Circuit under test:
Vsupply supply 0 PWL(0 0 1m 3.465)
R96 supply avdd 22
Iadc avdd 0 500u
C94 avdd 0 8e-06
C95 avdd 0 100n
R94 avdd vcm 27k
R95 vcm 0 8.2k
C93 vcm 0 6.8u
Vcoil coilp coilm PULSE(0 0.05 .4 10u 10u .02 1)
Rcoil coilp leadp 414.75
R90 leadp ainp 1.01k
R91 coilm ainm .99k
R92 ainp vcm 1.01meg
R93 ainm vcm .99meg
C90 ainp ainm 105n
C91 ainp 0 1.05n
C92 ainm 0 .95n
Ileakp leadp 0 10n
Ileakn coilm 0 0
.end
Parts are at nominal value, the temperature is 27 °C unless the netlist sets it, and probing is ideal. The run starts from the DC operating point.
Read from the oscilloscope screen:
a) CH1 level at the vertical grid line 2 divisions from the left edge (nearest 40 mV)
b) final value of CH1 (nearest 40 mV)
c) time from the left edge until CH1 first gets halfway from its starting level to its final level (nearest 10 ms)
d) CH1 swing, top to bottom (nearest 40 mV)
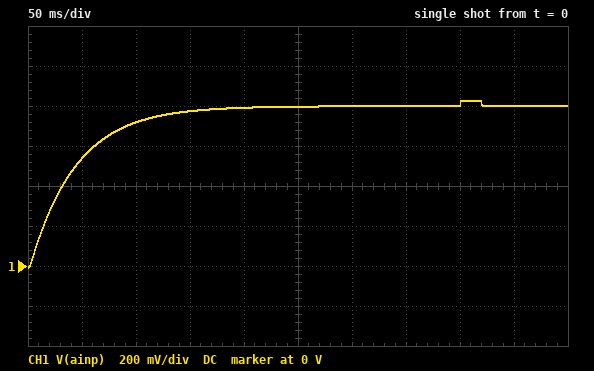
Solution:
720 mV
800 mV
30 ms
840 mV
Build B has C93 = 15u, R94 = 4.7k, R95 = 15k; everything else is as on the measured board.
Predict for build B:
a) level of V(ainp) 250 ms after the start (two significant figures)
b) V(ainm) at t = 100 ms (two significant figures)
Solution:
2.6 V
2.2 V
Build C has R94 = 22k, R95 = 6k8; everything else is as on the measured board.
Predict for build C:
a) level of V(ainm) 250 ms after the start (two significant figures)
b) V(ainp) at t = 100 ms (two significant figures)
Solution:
810 mV
760 mV
